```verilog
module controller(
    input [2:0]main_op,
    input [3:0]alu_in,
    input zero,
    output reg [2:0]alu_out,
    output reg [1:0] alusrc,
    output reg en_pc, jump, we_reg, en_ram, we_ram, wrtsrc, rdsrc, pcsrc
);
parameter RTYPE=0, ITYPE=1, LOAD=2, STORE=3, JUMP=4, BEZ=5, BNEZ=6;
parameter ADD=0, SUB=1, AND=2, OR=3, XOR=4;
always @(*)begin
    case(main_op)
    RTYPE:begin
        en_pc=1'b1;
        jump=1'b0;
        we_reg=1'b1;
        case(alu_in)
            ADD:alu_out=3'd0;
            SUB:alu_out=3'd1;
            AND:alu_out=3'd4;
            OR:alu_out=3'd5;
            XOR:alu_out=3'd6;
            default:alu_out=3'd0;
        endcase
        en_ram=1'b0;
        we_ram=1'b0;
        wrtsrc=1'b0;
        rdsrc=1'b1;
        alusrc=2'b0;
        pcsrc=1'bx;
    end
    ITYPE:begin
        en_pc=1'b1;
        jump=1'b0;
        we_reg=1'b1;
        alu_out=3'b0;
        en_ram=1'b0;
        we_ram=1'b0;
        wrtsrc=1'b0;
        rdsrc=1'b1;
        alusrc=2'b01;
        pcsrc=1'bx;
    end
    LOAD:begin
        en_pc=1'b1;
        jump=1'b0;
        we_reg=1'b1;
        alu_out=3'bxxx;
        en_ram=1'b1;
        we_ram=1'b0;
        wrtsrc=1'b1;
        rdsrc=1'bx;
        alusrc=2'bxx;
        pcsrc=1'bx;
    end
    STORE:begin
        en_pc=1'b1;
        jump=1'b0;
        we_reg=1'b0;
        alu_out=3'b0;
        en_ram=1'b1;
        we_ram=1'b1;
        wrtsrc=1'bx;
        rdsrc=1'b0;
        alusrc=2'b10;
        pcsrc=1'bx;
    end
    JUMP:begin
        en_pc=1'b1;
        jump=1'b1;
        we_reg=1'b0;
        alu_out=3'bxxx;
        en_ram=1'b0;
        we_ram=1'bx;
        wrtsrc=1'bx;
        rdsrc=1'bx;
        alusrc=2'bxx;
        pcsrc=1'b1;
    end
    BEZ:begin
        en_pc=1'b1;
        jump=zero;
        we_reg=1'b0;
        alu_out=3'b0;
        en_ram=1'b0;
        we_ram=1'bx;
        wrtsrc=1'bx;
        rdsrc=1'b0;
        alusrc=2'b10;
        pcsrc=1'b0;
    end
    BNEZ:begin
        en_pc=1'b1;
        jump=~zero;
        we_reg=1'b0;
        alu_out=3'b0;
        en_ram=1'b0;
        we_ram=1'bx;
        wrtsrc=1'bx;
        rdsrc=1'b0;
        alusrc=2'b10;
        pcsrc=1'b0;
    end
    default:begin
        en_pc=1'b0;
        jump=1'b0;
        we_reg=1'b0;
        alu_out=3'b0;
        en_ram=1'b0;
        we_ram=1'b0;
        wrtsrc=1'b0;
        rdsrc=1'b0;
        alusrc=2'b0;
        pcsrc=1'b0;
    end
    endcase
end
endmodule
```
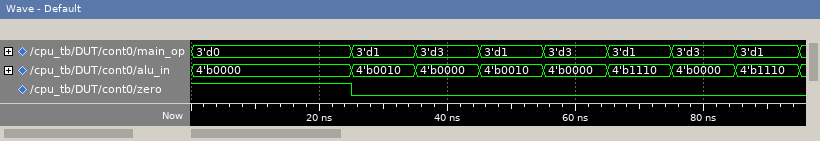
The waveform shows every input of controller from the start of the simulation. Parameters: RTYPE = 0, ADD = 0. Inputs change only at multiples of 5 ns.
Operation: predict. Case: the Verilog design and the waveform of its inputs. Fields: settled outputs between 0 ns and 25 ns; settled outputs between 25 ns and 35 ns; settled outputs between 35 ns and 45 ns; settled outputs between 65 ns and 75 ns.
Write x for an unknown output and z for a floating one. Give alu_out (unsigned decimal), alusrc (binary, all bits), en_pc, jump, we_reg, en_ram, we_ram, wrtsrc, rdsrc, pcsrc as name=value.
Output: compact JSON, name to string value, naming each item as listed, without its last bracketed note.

{"settled outputs between 0 ns and 25 ns": "alu_out=0, alusrc=00, en_pc=1, jump=0, we_reg=1, en_ram=0, we_ram=0, wrtsrc=0, rdsrc=1, pcsrc=x", "settled outputs between 25 ns and 35 ns": "alu_out=0, alusrc=01, en_pc=1, jump=0, we_reg=1, en_ram=0, we_ram=0, wrtsrc=0, rdsrc=1, pcsrc=x", "settled outputs between 35 ns and 45 ns": "alu_out=0, alusrc=10, en_pc=1, jump=0, we_reg=0, en_ram=1, we_ram=1, wrtsrc=x, rdsrc=0, pcsrc=x", "settled outputs between 65 ns and 75 ns": "alu_out=0, alusrc=01, en_pc=1, jump=0, we_reg=1, en_ram=0, we_ram=0, wrtsrc=0, rdsrc=1, pcsrc=x"}
